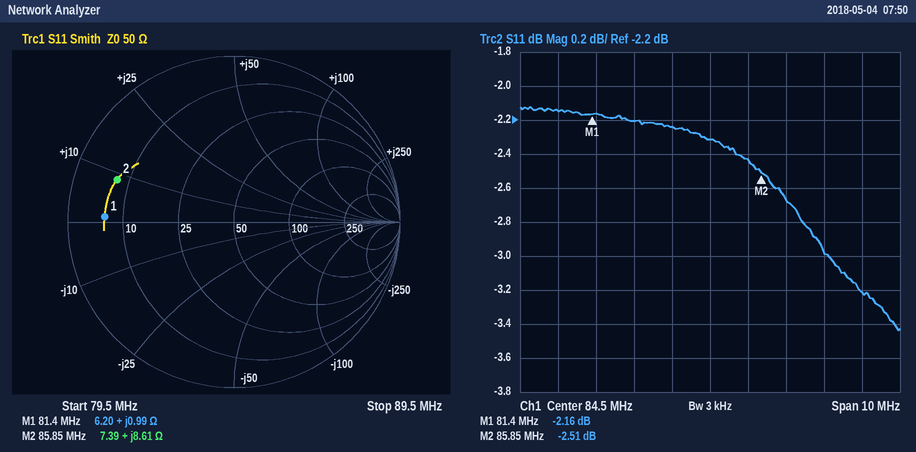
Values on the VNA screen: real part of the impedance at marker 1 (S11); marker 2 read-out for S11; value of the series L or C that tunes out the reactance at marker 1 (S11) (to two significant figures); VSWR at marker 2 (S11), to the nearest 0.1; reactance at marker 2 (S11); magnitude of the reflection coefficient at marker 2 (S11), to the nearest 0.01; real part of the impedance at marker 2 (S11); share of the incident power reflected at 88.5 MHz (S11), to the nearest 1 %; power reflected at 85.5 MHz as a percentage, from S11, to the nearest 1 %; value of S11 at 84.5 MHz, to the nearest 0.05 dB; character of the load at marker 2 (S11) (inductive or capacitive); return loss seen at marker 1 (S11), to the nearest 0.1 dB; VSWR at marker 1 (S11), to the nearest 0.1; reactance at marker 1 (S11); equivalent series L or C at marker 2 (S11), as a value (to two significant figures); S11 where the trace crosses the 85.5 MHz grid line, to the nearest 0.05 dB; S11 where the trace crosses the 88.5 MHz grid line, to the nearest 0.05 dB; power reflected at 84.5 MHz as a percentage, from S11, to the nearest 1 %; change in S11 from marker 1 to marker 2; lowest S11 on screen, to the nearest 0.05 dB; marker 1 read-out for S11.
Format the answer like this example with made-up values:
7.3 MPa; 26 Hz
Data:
6.20 Ω; -2.51 dB; 2.0 nF; 7.0; +8.61 Ω; 0.75; 7.39 Ω; 48 %; 57 %; -2.30 dB; inductive; 2.2 dB; 8.1; +0.99 Ω; 16 nH; -2.45 dB; -3.20 dB; 59 %; -0.35 dB; -3.45 dB; -2.16 dB
